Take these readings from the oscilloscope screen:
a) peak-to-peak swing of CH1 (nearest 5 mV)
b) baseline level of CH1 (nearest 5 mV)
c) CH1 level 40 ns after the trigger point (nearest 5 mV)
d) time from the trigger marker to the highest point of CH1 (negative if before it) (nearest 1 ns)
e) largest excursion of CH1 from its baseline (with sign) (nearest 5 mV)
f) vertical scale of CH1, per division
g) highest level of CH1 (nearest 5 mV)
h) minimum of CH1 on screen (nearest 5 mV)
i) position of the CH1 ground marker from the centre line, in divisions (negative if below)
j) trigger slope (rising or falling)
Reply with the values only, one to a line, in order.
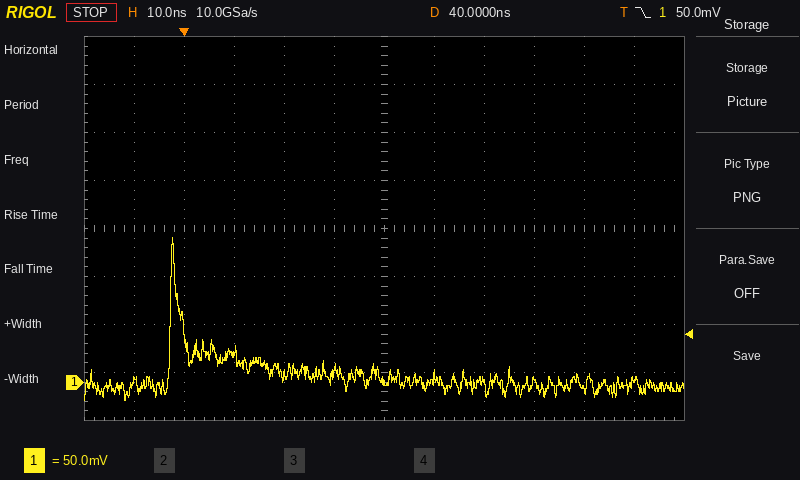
170 mV
0 mV
0 mV
-2 ns
+150 mV
50 mV
150 mV
-20 mV
-3.2 div
falling
